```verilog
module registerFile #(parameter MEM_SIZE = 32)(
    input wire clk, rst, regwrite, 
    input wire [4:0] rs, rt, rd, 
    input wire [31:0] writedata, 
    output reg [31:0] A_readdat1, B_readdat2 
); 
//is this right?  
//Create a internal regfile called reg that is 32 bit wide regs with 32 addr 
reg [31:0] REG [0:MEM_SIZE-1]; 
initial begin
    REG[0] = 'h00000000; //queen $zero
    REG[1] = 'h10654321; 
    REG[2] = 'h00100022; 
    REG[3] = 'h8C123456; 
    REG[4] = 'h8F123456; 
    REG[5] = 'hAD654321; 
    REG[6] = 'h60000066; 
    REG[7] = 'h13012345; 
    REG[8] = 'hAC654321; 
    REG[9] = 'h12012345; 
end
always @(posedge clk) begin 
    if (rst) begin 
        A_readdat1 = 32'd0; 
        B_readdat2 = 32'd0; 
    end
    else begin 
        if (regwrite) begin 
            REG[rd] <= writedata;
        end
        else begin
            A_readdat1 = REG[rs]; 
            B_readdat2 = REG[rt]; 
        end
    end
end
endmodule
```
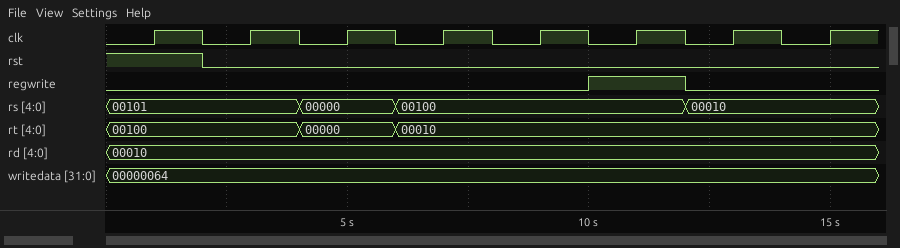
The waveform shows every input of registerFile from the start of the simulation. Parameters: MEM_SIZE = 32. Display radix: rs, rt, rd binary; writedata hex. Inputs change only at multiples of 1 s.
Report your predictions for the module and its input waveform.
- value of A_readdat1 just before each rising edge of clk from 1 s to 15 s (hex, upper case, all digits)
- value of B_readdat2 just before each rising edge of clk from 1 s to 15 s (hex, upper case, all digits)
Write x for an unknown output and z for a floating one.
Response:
x, 00000000, AD654321, 00000000, 8F123456, 8F123456, 8F123456, 00000064
x, 00000000, 8F123456, 00000000, 00100022, 00100022, 00100022, 00000064
